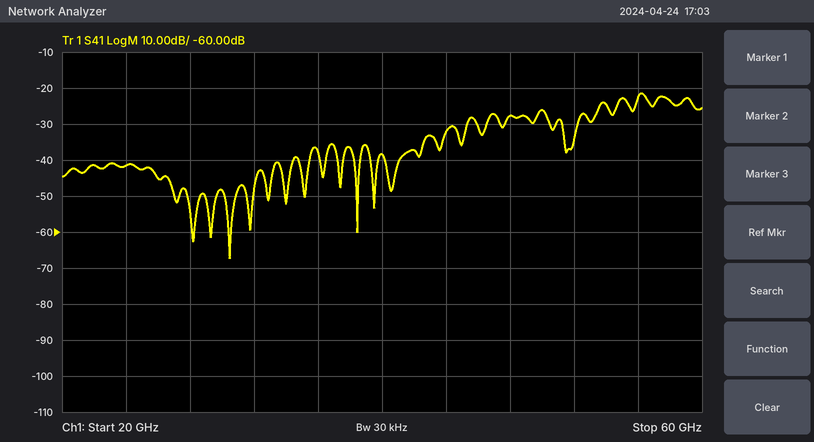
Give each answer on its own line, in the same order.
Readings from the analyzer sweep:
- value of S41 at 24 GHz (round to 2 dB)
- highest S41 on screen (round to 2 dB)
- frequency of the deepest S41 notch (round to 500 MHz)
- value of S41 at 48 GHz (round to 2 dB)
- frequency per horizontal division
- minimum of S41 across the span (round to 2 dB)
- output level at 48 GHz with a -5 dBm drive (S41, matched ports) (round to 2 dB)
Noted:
-42 dB
-22 dB
30.5 GHz
-28 dB
4 GHz
-68 dB
-32 dBm
